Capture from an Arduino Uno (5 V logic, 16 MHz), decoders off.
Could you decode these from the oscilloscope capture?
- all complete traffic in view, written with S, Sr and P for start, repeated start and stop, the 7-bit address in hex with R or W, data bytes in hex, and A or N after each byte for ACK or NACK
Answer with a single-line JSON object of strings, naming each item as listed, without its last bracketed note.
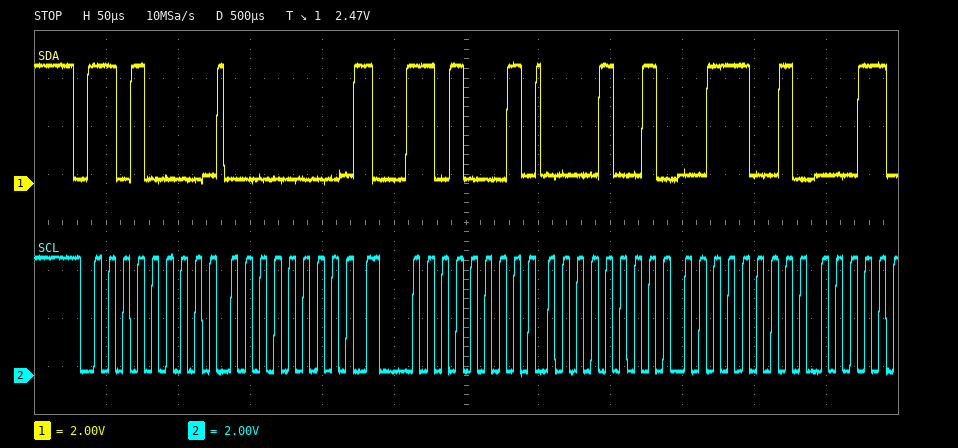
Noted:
{"all complete traffic in view, written with S, Sr and P for start, repeated start and stop, the 7-bit address in hex with R or W, data bytes in hex, and A or N after each byte for ACK or NACK": "S 68W A 00 A Sr 68R A 09 A 39 A"}
